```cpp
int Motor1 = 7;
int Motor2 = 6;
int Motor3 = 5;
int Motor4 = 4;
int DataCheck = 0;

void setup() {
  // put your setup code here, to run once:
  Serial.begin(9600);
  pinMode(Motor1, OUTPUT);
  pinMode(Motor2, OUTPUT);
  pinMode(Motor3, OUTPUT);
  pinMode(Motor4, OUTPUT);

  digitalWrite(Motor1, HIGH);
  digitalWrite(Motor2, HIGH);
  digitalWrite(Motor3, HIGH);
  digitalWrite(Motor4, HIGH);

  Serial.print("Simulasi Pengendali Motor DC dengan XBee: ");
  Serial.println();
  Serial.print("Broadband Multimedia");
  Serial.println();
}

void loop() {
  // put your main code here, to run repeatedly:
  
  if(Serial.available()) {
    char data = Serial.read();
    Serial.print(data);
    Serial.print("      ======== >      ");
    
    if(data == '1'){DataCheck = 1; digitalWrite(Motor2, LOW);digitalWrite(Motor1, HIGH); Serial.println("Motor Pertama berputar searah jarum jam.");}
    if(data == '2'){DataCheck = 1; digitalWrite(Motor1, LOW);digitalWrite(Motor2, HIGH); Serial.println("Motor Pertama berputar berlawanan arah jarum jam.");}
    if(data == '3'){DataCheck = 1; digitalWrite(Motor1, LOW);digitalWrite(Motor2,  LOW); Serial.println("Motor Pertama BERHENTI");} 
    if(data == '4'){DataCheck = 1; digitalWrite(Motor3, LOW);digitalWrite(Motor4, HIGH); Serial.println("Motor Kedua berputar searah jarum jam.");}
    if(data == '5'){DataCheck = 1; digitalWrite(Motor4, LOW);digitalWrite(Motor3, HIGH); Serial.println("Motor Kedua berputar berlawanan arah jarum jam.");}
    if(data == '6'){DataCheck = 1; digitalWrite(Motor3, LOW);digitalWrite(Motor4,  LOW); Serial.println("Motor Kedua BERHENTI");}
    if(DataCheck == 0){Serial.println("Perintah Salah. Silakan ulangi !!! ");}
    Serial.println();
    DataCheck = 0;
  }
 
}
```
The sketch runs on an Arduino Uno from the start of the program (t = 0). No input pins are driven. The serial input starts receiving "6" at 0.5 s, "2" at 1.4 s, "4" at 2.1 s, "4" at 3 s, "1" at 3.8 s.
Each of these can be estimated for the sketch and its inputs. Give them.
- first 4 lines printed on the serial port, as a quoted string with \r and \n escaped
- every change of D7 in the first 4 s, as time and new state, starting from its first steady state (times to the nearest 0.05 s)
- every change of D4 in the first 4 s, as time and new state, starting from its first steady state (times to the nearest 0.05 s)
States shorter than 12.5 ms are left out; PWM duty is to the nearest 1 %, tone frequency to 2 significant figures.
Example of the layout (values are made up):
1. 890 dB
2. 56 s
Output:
1. "Simulasi Pengendali Motor DC dengan XBee: \r\nBroadband Multimedia\r\n6      ======== >      Motor Kedua BERHENTI\r\n\r\n"
2. 0 s high; 1.4 s low; 3.8 s high
3. 0 s high; 0.5 s low; 2.1 s high
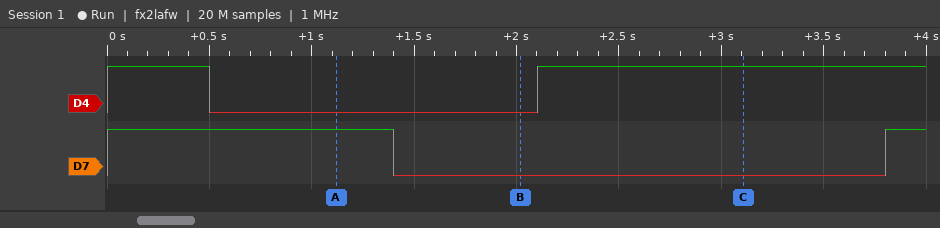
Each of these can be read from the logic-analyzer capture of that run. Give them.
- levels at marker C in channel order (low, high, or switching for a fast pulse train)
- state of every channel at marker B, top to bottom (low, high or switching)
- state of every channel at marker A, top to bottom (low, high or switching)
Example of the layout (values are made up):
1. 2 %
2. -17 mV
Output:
1. D4 high, D7 low
2. D4 low, D7 low
3. D4 low, D7 high
